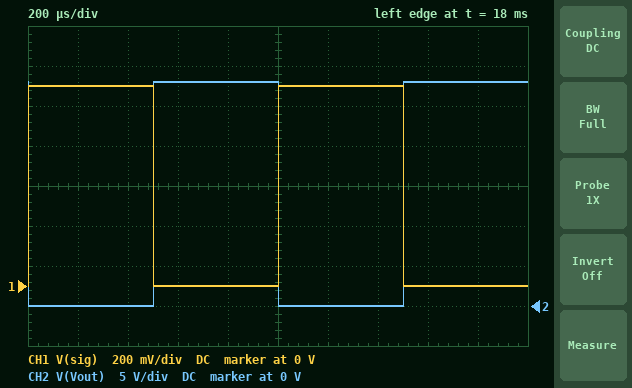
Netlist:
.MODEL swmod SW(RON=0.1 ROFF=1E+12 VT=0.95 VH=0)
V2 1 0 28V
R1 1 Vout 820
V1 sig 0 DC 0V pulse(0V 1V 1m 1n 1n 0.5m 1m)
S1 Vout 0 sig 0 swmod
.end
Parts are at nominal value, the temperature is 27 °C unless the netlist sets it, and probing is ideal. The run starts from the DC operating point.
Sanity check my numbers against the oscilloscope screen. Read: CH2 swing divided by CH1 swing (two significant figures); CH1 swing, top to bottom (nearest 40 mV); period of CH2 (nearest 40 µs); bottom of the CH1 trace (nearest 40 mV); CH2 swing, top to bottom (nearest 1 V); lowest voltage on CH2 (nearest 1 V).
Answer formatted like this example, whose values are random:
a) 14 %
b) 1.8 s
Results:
a) 28
b) 1.00 V
c) 1.00 ms
d) 0 V
e) 28 V
f) 0 V
